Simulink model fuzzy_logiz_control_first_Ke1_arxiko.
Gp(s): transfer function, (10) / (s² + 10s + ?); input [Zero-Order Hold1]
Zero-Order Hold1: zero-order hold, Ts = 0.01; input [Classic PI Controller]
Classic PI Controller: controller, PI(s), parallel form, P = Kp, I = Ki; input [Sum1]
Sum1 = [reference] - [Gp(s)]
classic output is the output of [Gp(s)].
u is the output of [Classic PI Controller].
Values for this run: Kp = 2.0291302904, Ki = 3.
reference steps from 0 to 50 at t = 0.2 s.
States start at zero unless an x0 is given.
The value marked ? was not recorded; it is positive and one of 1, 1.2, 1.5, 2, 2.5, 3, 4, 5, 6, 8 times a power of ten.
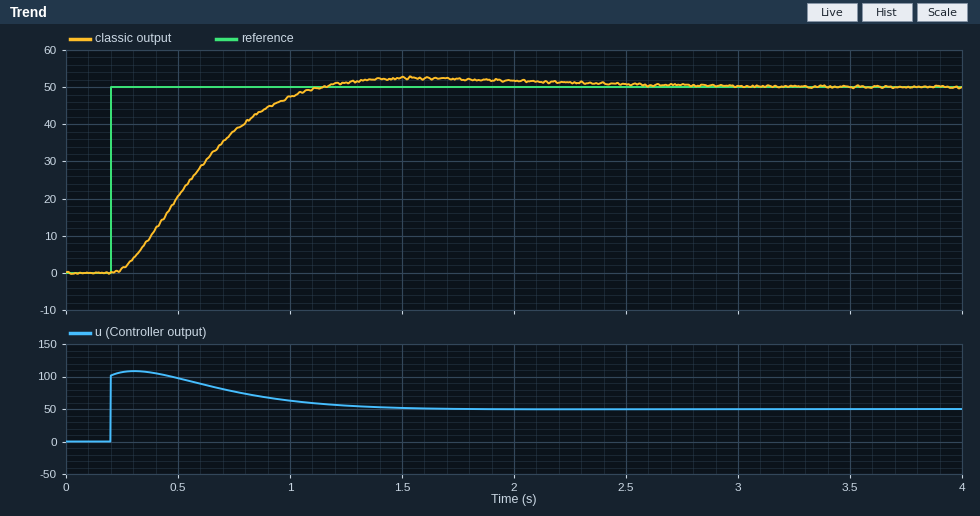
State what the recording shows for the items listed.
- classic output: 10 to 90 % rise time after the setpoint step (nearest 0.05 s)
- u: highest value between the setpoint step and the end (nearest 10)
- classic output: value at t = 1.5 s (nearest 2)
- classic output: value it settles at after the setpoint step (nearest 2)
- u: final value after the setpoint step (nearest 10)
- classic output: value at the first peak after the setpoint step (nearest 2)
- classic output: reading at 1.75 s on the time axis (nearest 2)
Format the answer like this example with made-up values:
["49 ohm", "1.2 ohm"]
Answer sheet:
["0.60 s", "110", "52", "50", "50", "52", "52"]
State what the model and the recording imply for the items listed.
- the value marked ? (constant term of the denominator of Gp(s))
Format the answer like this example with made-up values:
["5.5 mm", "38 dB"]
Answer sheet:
["10"]
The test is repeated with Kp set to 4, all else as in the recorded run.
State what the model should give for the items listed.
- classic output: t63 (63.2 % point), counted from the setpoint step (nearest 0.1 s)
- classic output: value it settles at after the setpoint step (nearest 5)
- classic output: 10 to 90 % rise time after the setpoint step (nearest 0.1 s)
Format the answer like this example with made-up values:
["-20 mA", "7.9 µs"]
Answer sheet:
["0.3 s", "50", "0.4 s"]
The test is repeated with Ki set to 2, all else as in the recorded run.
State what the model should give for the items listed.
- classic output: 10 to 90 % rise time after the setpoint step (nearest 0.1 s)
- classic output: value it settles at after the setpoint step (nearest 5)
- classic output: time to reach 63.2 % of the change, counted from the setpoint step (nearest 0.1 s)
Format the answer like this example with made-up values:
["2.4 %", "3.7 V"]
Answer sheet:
["0.8 s", "50", "0.5 s"]
